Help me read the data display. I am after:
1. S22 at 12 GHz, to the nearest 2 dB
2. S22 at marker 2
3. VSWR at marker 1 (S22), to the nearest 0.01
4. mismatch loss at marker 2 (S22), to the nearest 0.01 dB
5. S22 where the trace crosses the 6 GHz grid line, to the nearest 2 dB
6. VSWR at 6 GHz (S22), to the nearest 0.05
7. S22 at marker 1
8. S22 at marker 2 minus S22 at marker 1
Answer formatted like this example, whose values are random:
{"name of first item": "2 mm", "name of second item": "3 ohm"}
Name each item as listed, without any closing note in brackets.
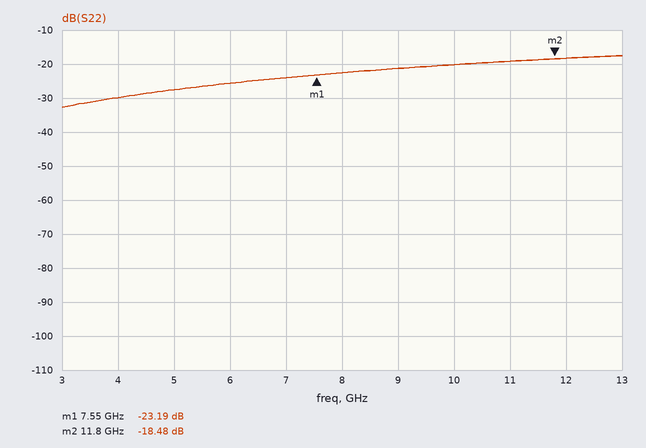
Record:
{"S22 at 12 GHz, to the nearest 2 dB": "-18 dB", "S22 at marker 2": "-18.48 dB", "VSWR at marker 1 (S22), to the nearest 0.01": "1.15", "mismatch loss at marker 2 (S22), to the nearest 0.01 dB": "0.06 dB", "S22 where the trace crosses the 6 GHz grid line, to the nearest 2 dB": "-26 dB", "VSWR at 6 GHz (S22), to the nearest 0.05": "1.10", "S22 at marker 1": "-23.19 dB", "S22 at marker 2 minus S22 at marker 1": "4.71 dB"}
